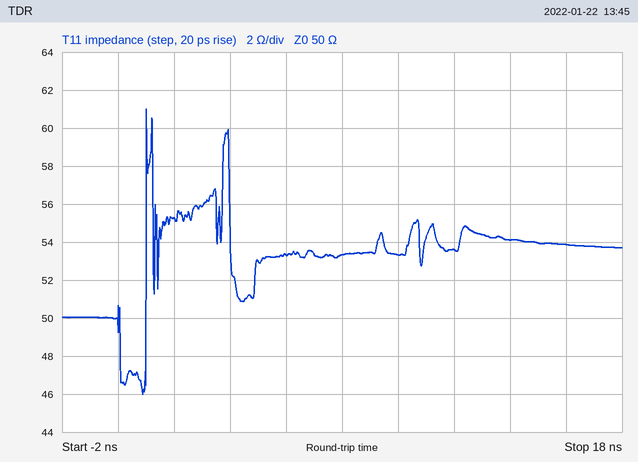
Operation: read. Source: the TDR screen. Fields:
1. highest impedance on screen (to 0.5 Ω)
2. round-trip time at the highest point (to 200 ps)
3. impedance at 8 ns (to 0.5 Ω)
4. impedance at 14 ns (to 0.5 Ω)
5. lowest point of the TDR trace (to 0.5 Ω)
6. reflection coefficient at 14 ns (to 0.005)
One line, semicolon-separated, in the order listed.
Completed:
61.0 Ω; 1.0 ns; 53.5 Ω; 54.0 Ω; 46.0 Ω; +0.040
